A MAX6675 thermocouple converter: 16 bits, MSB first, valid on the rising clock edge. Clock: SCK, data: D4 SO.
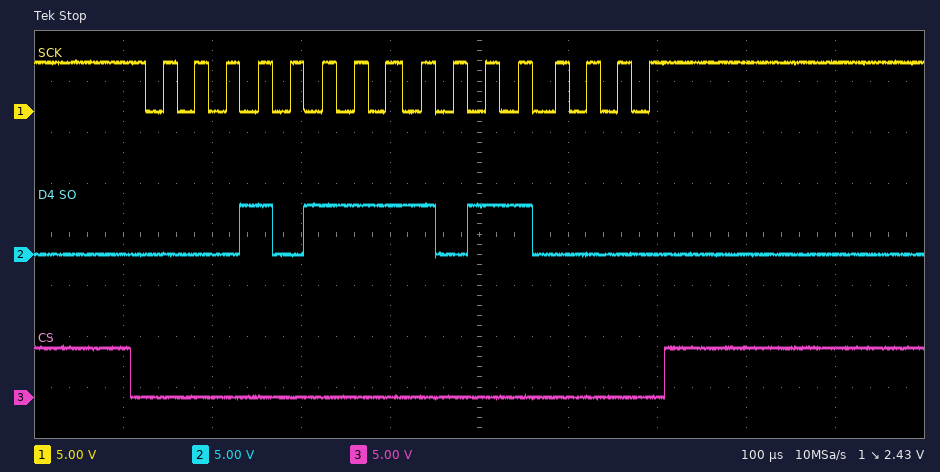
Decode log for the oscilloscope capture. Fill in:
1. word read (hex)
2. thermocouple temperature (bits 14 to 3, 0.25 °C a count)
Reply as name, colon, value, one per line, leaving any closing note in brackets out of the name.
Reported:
word read: 0x17B0
thermocouple temperature: 189.50 °C
